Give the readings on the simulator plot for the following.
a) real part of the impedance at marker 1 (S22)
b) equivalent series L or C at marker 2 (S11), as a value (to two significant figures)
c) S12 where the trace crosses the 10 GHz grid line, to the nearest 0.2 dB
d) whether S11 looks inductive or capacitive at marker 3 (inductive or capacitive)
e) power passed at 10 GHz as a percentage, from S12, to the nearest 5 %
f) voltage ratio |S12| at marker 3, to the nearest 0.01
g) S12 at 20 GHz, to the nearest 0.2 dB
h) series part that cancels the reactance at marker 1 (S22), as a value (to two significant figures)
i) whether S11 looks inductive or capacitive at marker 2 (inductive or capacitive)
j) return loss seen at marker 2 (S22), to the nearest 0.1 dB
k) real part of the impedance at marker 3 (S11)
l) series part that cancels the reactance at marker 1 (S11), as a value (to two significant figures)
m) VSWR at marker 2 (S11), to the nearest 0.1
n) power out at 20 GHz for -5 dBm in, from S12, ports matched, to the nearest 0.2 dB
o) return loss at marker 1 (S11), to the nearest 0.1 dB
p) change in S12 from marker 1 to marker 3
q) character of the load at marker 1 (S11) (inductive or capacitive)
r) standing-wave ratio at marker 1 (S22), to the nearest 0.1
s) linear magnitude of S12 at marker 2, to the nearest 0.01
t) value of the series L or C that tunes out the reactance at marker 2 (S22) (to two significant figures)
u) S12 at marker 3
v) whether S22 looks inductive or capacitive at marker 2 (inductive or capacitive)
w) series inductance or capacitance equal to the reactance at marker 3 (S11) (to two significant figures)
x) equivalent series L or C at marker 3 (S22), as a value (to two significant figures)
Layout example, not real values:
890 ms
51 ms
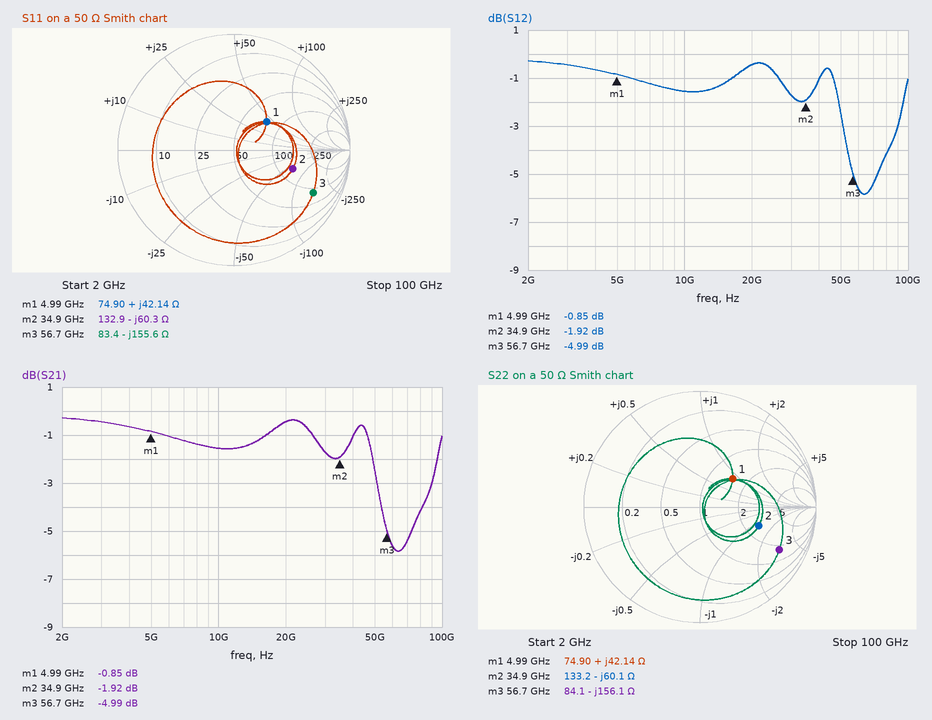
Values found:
74.90 Ω
76 fF
-1.6 dB
capacitive
70 %
0.56
-0.4 dB
760 fF
capacitive
5.5 dB
83.4 Ω
760 fF
3.3
-5.4 dBm
8.6 dB
-4.14 dB
inductive
2.2
0.80
270 pH
-4.99 dB
capacitive
18 fF
18 fF
